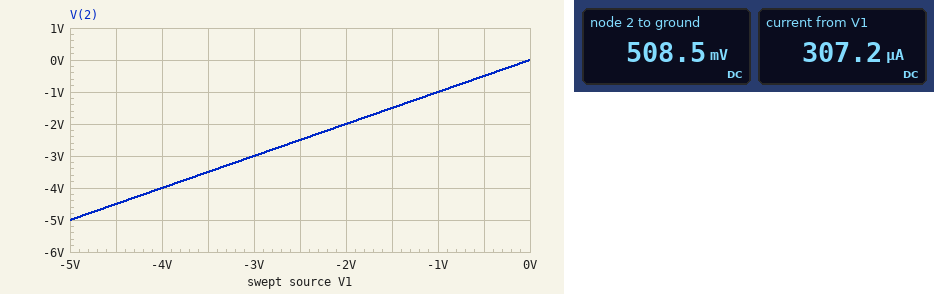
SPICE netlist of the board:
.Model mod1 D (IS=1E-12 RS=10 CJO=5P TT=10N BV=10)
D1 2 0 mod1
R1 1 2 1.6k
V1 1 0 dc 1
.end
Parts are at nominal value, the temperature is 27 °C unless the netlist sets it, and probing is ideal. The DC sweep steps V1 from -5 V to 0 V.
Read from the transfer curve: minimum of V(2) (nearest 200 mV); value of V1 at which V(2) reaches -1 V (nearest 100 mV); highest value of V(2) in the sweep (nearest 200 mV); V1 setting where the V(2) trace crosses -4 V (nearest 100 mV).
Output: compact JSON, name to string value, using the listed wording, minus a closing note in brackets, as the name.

{"minimum of V(2)": "-5.0 V", "value of V1 at which V(2) reaches -1 V": "-1.0 V", "highest value of V(2) in the sweep": "0 V", "V1 setting where the V(2) trace crosses -4 V": "-4.0 V"}
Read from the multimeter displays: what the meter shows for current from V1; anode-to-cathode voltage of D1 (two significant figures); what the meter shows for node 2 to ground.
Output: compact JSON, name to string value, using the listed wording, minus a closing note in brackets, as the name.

{"what the meter shows for current from V1": "307.2 µA", "anode-to-cathode voltage of D1": "510 mV", "what the meter shows for node 2 to ground": "508.5 mV"}
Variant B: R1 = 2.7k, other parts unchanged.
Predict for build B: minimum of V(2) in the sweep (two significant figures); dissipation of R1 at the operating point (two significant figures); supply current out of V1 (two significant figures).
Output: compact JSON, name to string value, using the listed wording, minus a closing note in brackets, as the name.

{"minimum of V(2) in the sweep": "-5.0 V", "dissipation of R1 at the operating point": "95 µW", "supply current out of V1": "190 µA"}
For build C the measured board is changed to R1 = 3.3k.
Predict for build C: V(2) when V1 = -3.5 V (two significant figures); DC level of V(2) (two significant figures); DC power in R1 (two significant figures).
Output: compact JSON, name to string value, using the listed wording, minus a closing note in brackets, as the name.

{"V(2) when V1 = -3.5 V": "-3.5 V", "DC level of V(2)": "490 mV", "DC power in R1": "79 µW"}
